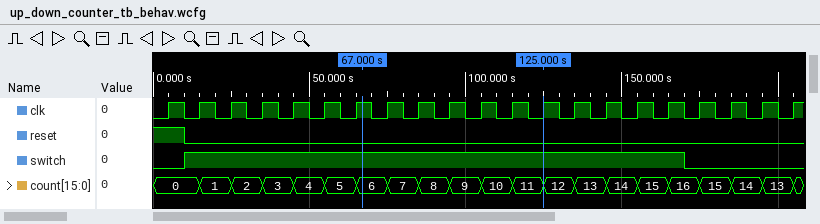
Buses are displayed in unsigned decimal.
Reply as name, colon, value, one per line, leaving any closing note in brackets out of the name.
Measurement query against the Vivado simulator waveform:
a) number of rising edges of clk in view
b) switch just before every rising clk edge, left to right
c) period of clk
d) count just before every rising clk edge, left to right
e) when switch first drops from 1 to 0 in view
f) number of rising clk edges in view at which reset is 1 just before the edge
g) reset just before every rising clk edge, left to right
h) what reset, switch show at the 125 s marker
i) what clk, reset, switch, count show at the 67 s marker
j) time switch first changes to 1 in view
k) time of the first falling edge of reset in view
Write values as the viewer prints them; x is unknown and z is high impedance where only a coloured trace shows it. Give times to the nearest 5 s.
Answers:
number of rising edges of clk in view: 21
switch just before every rising clk edge, left to right: 0 1 1 1 1 1 1 1 1 1 1 1 1 1 1 1 1 0 0 0 0
period of clk: 10 s
count just before every rising clk edge, left to right: 0, 0, 1, 2, 3, 4, 5, 6, 7, 8, 9, 10, 11, 12, 13, 14, 15, 16, 15, 14, 13
when switch first drops from 1 to 0 in view: 170 s
number of rising clk edges in view at which reset is 1 just before the edge: 1
reset just before every rising clk edge, left to right: 1 0 0 0 0 0 0 0 0 0 0 0 0 0 0 0 0 0 0 0 0
what reset, switch show at the 125 s marker: reset=0, switch=1
what clk, reset, switch, count show at the 67 s marker: clk=1, reset=0, switch=1, count=6
time switch first changes to 1 in view: 10 s
time of the first falling edge of reset in view: 10 s
